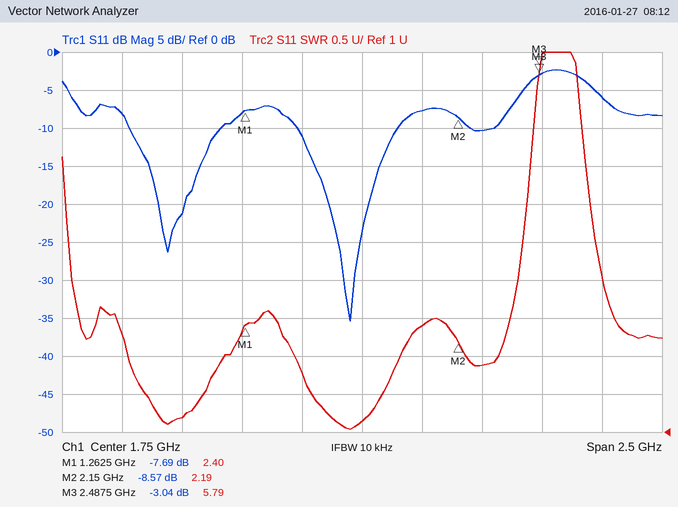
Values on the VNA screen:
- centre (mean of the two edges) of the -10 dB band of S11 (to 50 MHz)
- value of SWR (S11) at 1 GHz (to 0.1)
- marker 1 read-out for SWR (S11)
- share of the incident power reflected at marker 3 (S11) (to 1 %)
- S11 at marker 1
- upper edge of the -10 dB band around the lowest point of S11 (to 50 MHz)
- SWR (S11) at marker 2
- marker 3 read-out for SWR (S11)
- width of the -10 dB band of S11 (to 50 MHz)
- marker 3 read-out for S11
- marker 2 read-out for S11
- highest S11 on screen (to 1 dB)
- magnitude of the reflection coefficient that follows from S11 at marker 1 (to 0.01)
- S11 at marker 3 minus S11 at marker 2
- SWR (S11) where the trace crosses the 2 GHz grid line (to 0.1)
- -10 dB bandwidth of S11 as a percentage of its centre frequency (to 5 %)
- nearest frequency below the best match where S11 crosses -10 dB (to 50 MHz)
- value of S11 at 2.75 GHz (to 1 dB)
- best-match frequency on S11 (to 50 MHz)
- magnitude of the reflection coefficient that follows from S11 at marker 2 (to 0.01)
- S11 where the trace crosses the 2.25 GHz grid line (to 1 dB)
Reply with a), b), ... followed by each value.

a) 1.70 GHz
b) 1.2
c) 2.40
d) 50 %
e) -7.69 dB
f) 1.90 GHz
g) 2.19
h) 5.79
i) 400 MHz
j) -3.04 dB
k) -8.57 dB
l) -2 dB
m) 0.41
n) 5.53 dB
o) 2.4
p) 25 %
q) 1.50 GHz
r) -6 dB
s) 1.70 GHz
t) 0.37
u) -10 dB
